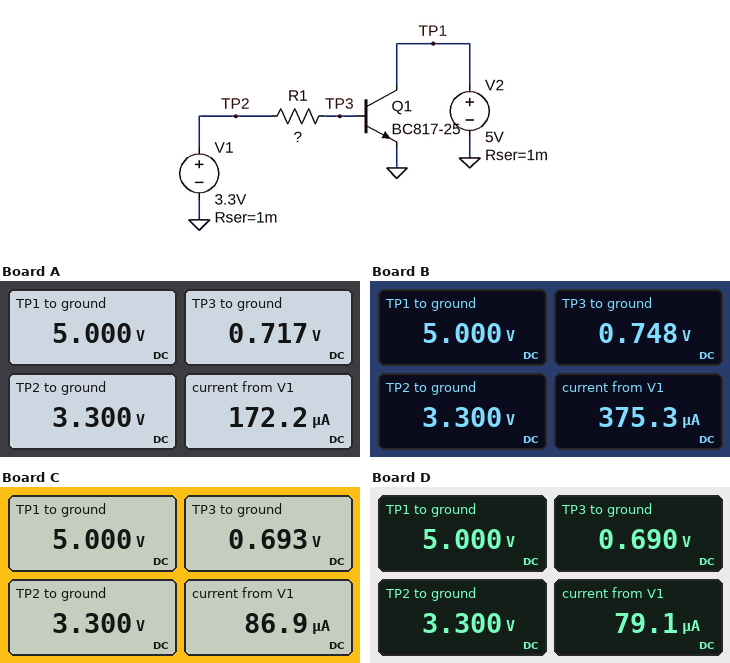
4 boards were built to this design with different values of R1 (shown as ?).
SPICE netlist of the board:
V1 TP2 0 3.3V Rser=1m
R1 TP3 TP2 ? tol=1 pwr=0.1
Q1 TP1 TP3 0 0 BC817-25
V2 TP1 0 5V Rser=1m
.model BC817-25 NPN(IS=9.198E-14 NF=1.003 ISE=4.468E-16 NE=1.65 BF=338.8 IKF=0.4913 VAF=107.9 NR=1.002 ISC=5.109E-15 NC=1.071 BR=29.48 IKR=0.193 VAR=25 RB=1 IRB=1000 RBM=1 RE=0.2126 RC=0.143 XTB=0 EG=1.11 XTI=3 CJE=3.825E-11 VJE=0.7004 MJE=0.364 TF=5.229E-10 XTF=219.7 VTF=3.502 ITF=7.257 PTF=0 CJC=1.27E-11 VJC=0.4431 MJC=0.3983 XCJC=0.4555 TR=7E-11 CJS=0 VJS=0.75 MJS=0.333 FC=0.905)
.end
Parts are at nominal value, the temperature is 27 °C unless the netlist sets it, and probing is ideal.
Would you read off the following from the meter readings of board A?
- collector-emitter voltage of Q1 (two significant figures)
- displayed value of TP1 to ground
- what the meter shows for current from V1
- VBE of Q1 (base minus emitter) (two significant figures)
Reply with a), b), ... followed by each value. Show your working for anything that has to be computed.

a) 5 V = 5.0 V
b) 5.000 V
c) 172.2 µA
d) 717 mV = 720 mV
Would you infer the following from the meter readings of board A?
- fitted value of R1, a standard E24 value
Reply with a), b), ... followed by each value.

a) 15 kΩ
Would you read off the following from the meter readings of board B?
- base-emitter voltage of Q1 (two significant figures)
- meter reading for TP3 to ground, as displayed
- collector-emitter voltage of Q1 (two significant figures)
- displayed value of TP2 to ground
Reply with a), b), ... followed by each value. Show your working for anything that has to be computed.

a) 748 mV = 750 mV
b) 0.748 V
c) 5 V = 5.0 V
d) 3.300 V
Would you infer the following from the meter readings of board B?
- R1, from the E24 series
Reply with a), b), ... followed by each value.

a) 6.8 kΩ
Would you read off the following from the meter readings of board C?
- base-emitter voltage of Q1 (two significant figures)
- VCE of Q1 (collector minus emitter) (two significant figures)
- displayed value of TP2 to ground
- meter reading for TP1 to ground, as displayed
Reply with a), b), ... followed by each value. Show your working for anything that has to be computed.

a) 693 mV = 690 mV
b) 5 V = 5.0 V
c) 3.300 V
d) 5.000 V
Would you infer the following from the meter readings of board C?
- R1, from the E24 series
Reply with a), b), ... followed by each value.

a) 30 kΩ
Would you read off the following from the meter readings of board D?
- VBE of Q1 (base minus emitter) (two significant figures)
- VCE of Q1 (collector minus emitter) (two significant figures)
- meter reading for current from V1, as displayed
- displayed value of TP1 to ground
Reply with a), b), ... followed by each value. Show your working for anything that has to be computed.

a) 690 mV = 690 mV
b) 5 V = 5.0 V
c) 79.1 µA
d) 5.000 V
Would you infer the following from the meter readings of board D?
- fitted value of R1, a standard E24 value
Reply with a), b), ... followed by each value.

a) 33 kΩ
